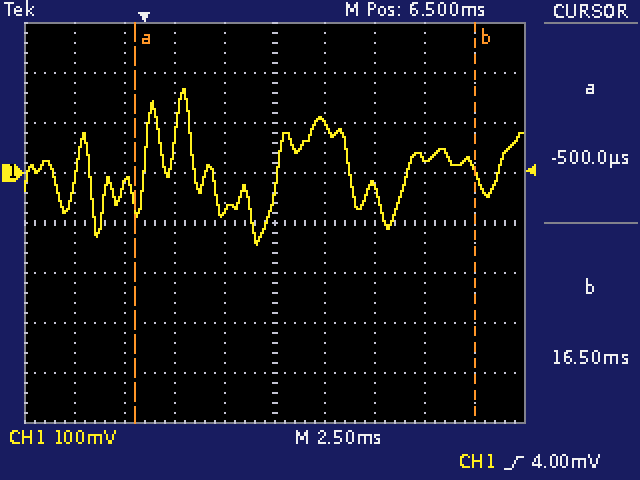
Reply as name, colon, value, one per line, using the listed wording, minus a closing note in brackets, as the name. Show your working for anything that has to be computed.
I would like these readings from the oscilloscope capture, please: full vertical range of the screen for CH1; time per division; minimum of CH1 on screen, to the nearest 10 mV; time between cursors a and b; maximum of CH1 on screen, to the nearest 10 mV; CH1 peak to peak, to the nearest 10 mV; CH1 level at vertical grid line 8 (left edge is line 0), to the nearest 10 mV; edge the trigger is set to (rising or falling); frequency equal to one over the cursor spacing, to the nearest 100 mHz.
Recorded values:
full vertical range of the screen for CH1: 800 mV
time per division: 2.5 ms
minimum of CH1 on screen, to the nearest 10 mV: -140 mV
time between cursors a and b: 16.5 ms − (-500 µs) = 17.00 ms
maximum of CH1 on screen, to the nearest 10 mV: 170 mV
CH1 peak to peak, to the nearest 10 mV: 170 mV − (-140 mV) = 310 mV
CH1 level at vertical grid line 8 (left edge is line 0), to the nearest 10 mV: 30 mV
edge the trigger is set to: rising
frequency equal to one over the cursor spacing, to the nearest 100 mHz: 1 / 17.00 ms ≈ 58.8 Hz
